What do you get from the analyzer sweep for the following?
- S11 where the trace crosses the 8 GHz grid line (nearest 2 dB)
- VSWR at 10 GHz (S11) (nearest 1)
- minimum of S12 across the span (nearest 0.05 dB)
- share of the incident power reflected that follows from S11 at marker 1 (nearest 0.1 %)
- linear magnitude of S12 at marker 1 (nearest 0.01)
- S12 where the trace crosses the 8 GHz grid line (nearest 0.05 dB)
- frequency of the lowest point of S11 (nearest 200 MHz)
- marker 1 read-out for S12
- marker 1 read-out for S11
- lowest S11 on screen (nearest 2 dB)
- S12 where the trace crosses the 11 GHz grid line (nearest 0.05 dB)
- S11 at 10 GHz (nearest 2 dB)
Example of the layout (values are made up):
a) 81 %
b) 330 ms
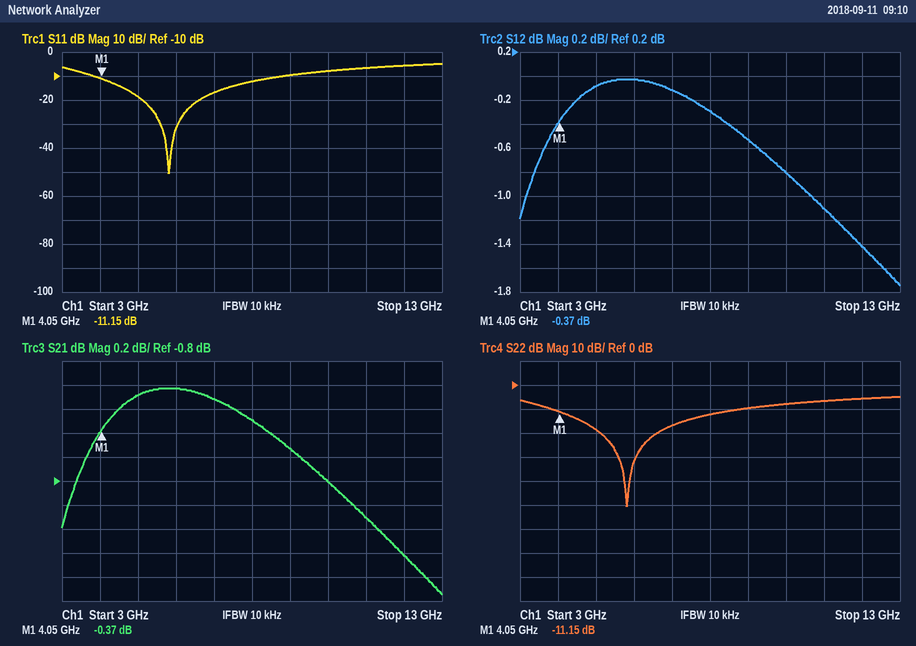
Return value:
a) -12 dB
b) 2
c) -1.75 dB
d) 7.7 %
e) 0.96
f) -0.30 dB
g) 5.8 GHz
h) -0.37 dB
i) -11.15 dB
j) -50 dB
k) -1.10 dB
l) -8 dB
